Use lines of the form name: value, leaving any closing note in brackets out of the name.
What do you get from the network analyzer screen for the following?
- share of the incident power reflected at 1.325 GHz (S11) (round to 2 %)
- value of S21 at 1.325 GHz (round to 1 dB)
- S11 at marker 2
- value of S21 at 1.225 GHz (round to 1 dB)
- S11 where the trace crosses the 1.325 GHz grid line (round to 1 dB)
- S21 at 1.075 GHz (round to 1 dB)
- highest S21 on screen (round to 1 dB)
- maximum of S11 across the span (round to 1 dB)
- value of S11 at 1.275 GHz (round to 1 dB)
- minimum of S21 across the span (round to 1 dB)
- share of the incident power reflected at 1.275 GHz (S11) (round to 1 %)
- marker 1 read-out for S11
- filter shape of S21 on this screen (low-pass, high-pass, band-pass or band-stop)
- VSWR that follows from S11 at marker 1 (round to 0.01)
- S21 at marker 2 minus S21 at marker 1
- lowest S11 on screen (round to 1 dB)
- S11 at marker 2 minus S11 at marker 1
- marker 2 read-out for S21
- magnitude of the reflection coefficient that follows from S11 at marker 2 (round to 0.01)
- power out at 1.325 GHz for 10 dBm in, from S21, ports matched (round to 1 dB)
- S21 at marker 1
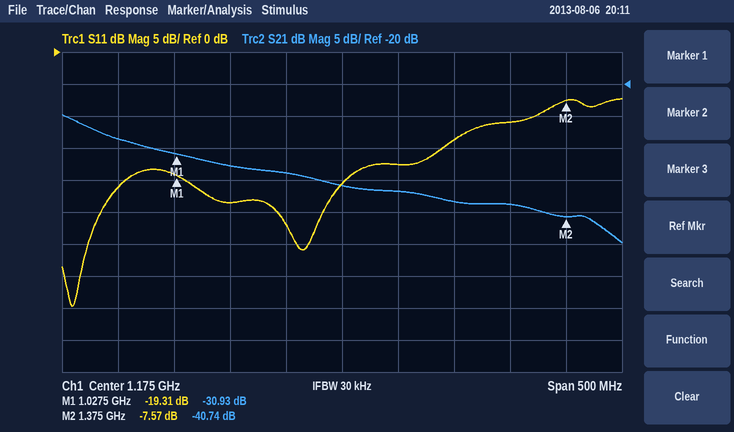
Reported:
share of the incident power reflected at 1.325 GHz (S11): 8 %
value of S21 at 1.325 GHz: -39 dB
S11 at marker 2: -7.57 dB
value of S21 at 1.225 GHz: -37 dB
S11 where the trace crosses the 1.325 GHz grid line: -11 dB
S21 at 1.075 GHz: -33 dB
highest S21 on screen: -25 dB
maximum of S11 across the span: -7 dB
value of S11 at 1.275 GHz: -14 dB
minimum of S21 across the span: -45 dB
share of the incident power reflected at 1.275 GHz (S11): 4 %
marker 1 read-out for S11: -19.31 dB
filter shape of S21 on this screen: low-pass
VSWR that follows from S11 at marker 1: 1.24
S21 at marker 2 minus S21 at marker 1: -9.81 dB
lowest S11 on screen: -40 dB
S11 at marker 2 minus S11 at marker 1: 11.74 dB
marker 2 read-out for S21: -40.74 dB
magnitude of the reflection coefficient that follows from S11 at marker 2: 0.42
power out at 1.325 GHz for 10 dBm in, from S21, ports matched: -29 dBm
S21 at marker 1: -30.93 dB
